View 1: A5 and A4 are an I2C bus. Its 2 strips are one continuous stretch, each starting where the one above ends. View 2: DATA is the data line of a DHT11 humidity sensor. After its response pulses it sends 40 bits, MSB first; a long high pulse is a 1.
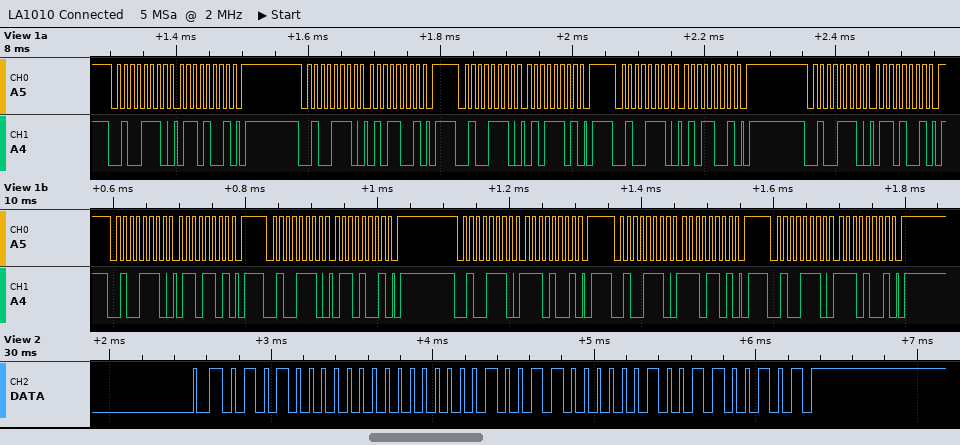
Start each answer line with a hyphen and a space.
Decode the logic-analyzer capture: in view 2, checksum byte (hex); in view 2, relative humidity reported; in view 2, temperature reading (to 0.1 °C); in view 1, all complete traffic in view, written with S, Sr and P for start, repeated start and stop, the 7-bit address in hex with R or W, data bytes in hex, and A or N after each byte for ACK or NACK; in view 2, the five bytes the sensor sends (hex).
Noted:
- 0x65
- 80 %
- 19.2 °C
- S 27W A 69 A P S 27W A 59 A P S 27W A 5D A P S 27W A 59 A P S 27W A 69 A P S 27W A 6D A P S 27W A 69 A P S 27W A E9 A P S 27W A ED A P S 27W A E9 A P
- 50 00 13 02 65
